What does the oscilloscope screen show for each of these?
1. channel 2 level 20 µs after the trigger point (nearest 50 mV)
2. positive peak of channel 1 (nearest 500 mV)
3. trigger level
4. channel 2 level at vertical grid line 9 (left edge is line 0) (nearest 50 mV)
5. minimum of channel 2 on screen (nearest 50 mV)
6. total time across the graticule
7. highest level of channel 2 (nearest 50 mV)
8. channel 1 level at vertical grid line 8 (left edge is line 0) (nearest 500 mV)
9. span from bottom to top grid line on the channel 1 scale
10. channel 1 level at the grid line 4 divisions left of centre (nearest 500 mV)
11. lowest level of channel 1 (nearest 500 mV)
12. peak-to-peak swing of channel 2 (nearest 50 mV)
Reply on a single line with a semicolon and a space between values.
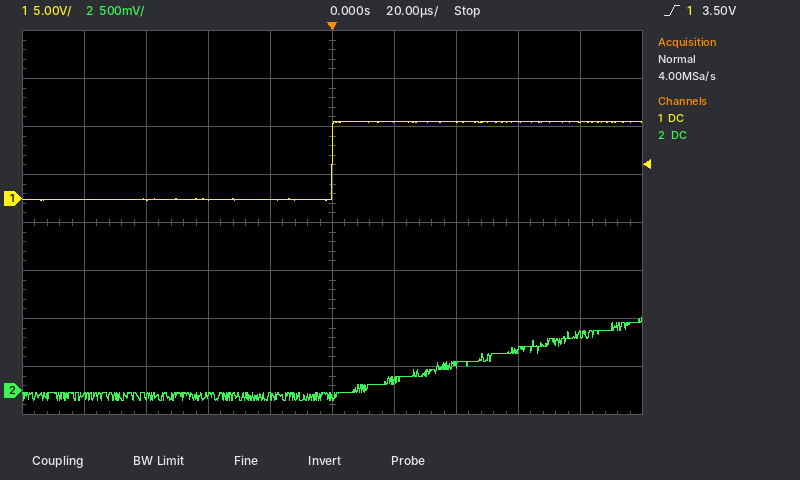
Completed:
100 mV; 8.0 V; 3.50 V; 600 mV; -100 mV; 200 µs; 750 mV; 8.0 V; 40 V; 0.0 V; 0.0 V; 850 mV
